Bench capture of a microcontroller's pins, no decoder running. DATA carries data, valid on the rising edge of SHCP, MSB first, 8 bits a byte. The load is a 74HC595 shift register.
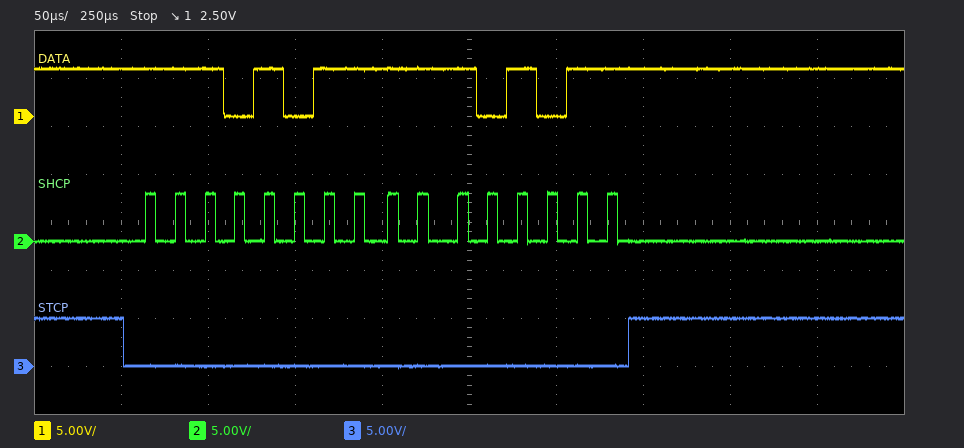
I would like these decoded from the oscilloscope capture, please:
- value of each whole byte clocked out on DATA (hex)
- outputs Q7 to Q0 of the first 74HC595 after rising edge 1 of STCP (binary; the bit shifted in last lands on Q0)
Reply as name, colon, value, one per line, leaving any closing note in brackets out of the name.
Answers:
value of each whole byte clocked out on DATA: EB EB
outputs Q7 to Q0 of the first 74HC595 after rising edge 1 of STCP: 11101011
